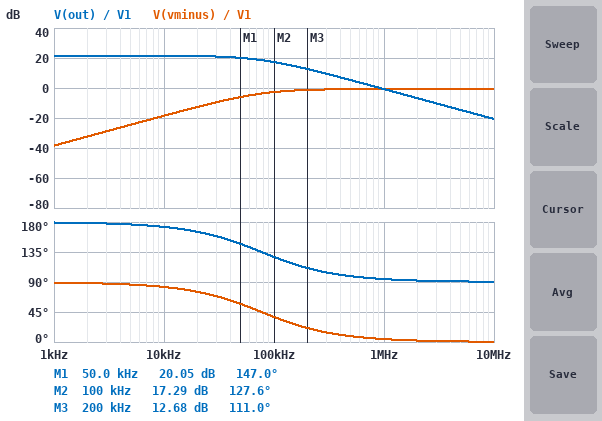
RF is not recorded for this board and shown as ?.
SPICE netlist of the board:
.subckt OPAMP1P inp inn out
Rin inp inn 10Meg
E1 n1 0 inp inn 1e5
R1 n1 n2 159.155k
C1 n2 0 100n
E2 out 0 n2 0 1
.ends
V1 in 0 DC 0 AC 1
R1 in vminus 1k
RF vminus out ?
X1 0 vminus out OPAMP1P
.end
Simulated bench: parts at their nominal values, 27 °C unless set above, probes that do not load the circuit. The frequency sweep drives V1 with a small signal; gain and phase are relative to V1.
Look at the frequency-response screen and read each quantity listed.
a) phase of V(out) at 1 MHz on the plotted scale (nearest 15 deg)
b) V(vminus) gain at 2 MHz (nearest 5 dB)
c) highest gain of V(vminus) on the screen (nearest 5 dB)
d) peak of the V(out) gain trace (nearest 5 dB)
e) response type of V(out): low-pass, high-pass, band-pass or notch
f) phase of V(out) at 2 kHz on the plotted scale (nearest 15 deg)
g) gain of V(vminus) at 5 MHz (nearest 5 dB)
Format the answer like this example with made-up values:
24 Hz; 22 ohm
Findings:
90 deg; 0 dB; 0 dB; 20 dB; low-pass; 180 deg; 0 dB
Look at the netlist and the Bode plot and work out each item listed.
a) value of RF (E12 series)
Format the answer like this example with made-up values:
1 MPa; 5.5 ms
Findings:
12 kΩ
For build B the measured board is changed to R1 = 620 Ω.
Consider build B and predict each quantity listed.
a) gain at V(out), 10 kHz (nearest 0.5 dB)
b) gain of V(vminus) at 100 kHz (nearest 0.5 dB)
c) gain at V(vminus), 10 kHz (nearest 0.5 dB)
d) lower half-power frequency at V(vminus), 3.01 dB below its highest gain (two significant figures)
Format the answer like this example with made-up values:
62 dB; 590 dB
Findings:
25.5 dB; -1.5 dB; -14.5 dB; 49 kHz
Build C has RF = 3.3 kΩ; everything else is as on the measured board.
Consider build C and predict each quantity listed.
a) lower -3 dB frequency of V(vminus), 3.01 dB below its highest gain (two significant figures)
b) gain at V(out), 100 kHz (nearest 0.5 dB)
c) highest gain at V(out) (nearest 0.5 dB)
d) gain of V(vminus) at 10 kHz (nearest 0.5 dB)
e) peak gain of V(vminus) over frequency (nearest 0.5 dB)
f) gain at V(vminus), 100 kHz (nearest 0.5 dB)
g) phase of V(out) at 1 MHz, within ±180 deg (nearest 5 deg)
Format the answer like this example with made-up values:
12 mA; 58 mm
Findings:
230 kHz; 9.5 dB; 10.5 dB; -29.5 dB; -2.5 dB; -10.5 dB; 105 deg
